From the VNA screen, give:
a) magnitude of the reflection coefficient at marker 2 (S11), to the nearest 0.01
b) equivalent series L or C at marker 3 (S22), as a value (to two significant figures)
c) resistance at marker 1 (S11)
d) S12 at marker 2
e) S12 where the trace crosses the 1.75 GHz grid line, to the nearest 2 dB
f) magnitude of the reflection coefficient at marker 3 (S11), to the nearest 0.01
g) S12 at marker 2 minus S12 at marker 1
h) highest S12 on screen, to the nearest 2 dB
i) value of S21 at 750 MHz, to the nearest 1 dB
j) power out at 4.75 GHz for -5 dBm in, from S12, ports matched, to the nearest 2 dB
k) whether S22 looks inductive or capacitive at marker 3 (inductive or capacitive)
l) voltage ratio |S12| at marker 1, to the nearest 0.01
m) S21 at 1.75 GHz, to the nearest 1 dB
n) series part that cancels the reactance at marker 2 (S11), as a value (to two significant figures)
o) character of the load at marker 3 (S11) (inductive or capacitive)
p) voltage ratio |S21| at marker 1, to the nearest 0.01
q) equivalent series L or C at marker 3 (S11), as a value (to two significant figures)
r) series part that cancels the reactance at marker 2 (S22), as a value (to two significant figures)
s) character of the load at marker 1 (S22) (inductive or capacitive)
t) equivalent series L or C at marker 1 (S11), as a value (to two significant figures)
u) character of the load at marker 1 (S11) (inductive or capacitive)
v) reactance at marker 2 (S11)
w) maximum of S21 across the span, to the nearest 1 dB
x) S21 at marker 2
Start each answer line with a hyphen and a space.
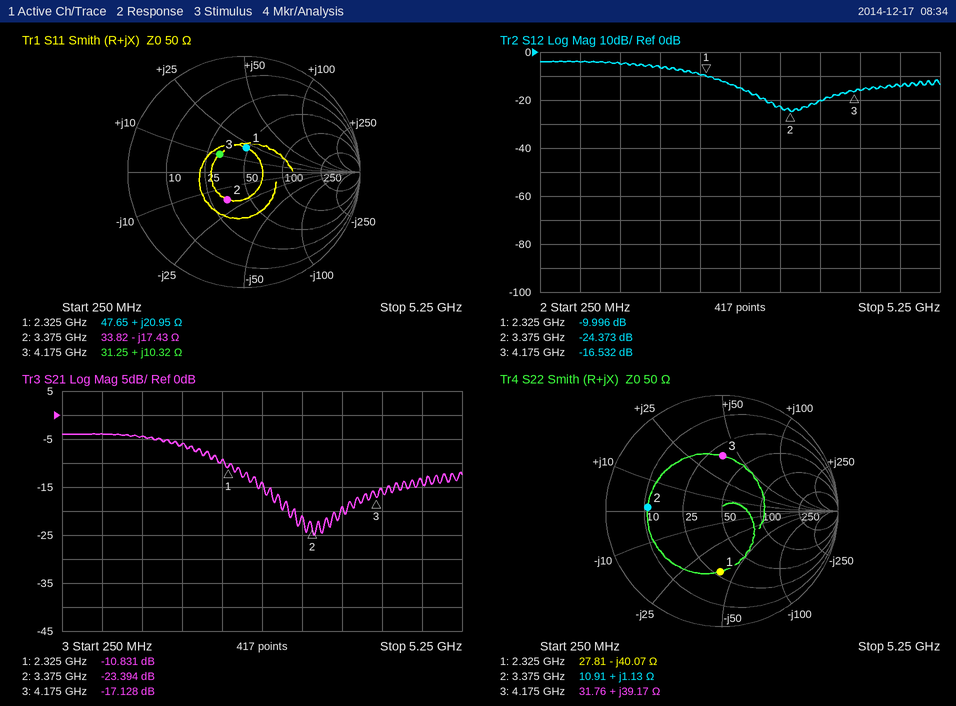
- 0.28
- 1.5 nH
- 47.65 Ω
- -24.373 dB
- -6 dB
- 0.26
- -14.377 dB
- -4 dB
- -4 dB
- -20 dBm
- inductive
- 0.32
- -6 dB
- 820 pH
- inductive
- 0.29
- 390 pH
- 42 pF
- capacitive
- 1.4 nH
- inductive
- -17.43 Ω
- -4 dB
- -23.394 dB
